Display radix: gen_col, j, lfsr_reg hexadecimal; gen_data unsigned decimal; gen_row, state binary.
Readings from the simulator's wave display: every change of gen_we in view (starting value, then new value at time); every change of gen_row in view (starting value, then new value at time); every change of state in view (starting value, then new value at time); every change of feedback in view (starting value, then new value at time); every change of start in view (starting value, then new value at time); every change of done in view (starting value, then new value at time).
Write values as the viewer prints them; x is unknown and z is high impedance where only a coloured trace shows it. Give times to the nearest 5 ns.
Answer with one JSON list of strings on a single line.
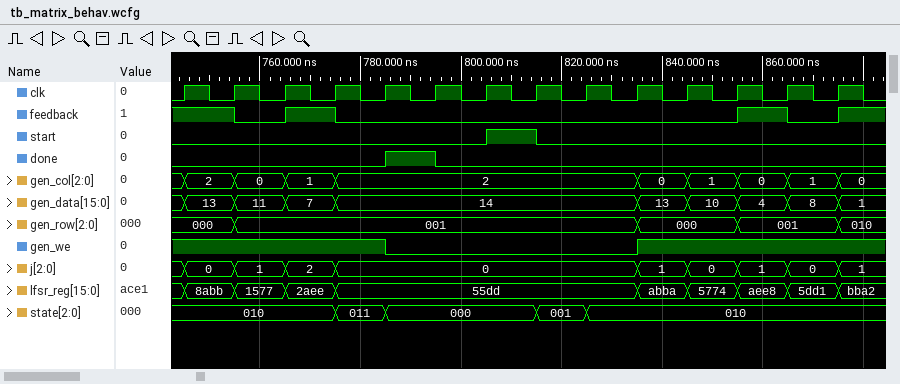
["1, 0 at 785 ns, 1 at 835 ns", "000, 001 at 755 ns, 000 at 835 ns, 001 at 855 ns, 010 at 875 ns", "010, 011 at 775 ns, 000 at 785 ns, 001 at 815 ns, 010 at 825 ns", "1, 0 at 755 ns, 1 at 765 ns, 0 at 775 ns, 1 at 855 ns, 0 at 865 ns, 1 at 875 ns", "0, 1 at 805 ns, 0 at 815 ns", "0, 1 at 785 ns, 0 at 795 ns"]
